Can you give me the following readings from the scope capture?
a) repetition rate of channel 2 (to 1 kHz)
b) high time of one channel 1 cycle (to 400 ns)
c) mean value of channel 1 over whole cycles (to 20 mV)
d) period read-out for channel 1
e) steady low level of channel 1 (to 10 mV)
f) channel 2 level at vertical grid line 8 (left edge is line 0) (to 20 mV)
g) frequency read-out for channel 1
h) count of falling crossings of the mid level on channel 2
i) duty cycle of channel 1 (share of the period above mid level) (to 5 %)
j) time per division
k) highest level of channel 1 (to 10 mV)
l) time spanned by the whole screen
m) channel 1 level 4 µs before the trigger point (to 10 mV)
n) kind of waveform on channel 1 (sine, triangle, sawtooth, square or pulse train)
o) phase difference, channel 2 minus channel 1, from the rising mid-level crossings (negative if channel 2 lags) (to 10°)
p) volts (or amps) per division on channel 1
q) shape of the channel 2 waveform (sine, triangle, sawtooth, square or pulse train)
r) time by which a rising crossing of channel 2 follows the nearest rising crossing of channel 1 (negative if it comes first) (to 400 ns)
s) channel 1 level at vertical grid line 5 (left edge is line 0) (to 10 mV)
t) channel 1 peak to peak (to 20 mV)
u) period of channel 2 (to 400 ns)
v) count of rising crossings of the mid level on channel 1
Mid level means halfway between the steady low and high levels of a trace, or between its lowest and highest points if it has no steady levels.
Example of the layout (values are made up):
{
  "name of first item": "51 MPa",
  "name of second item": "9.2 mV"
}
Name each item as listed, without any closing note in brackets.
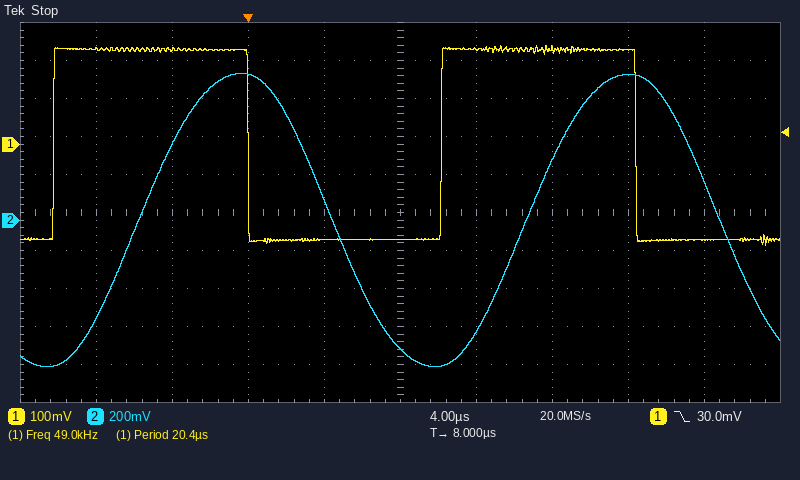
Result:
{
  "repetition rate of channel 2": "49 kHz",
  "high time of one channel 1 cycle": "10.4 µs",
  "mean value of channel 1 over whole cycles": "0 mV",
  "period read-out for channel 1": "20.4 µs",
  "steady low level of channel 1": "-250 mV",
  "channel 2 level at vertical grid line 8 (left edge is line 0)": "760 mV",
  "frequency read-out for channel 1": "49.0 kHz",
  "count of falling crossings of the mid level on channel 2": "2",
  "duty cycle of channel 1 (share of the period above mid level)": "50 %",
  "time per division": "4 µs",
  "highest level of channel 1": "260 mV",
  "time spanned by the whole screen": "40 µs",
  "channel 1 level 4 µs before the trigger point": "250 mV",
  "kind of waveform on channel 1": "square",
  "phase difference, channel 2 minus channel 1, from the rising mid-level crossings (negative if channel 2 lags)": "-80°",
  "volts (or amps) per division on channel 1": "100 mV",
  "shape of the channel 2 waveform": "sine",
  "time by which a rising crossing of channel 2 follows the nearest rising crossing of channel 1 (negative if it comes first)": "+4.4 µs",
  "channel 1 level at vertical grid line 5 (left edge is line 0)": "-250 mV",
  "channel 1 peak to peak": "520 mV",
  "period of channel 2": "20.4 µs",
  "count of rising crossings of the mid level on channel 1": "2"
}
